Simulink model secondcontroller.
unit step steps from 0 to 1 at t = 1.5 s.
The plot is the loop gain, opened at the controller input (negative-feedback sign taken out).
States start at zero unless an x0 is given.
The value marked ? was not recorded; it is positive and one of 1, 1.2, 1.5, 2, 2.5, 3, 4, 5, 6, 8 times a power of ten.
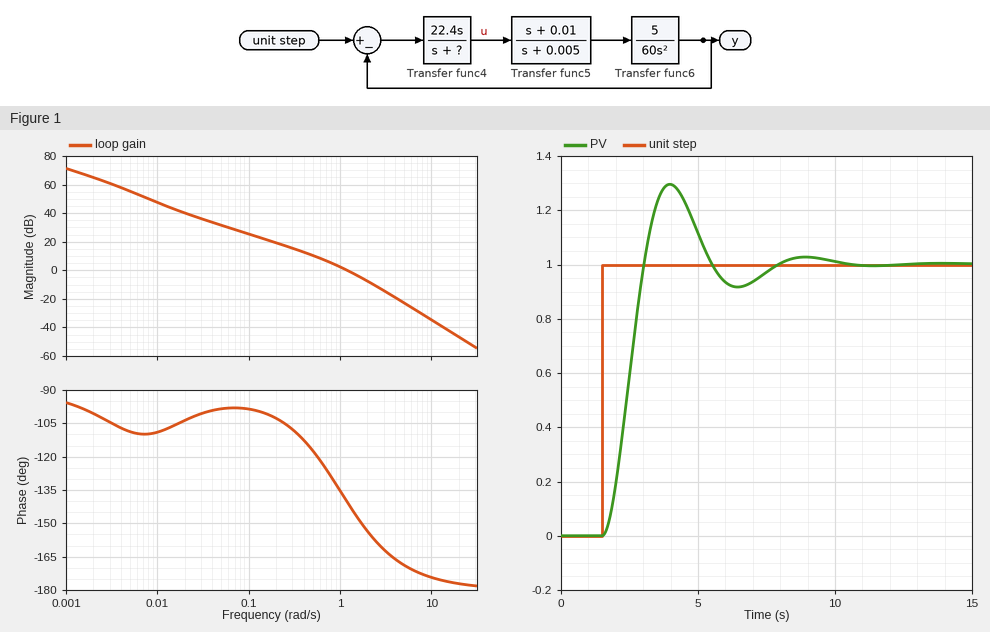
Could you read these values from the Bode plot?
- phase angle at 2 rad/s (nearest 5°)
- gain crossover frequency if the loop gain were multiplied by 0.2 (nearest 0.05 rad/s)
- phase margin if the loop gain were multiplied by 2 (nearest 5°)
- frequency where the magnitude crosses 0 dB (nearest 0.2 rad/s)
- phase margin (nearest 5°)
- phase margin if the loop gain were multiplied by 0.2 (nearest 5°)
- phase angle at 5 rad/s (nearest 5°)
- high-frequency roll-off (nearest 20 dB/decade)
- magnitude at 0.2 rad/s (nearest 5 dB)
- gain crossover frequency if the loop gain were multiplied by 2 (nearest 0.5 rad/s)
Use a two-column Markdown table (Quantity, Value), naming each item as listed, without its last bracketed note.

| Quantity | Value |
|---|---|
| phase angle at 2 rad/s | -155° |
| gain crossover frequency if the loop gain were multiplied by 0.2 | 0.35 rad/s |
| phase margin if the loop gain were multiplied by 2 | 30° |
| frequency where the magnitude crosses 0 dB | 1.2 rad/s |
| phase margin | 40° |
| phase margin if the loop gain were multiplied by 0.2 | 70° |
| phase angle at 5 rad/s | -170° |
| high-frequency roll-off | -40 dB/decade |
| magnitude at 0.2 rad/s | 20 dB |
| gain crossover frequency if the loop gain were multiplied by 2 | 2.0 rad/s |
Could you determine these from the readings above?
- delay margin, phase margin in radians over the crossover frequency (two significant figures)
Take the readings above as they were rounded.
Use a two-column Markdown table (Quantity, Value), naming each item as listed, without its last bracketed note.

| Quantity | Value |
|---|---|
| delay margin, phase margin in radians over the crossover frequency | 0.58 s |
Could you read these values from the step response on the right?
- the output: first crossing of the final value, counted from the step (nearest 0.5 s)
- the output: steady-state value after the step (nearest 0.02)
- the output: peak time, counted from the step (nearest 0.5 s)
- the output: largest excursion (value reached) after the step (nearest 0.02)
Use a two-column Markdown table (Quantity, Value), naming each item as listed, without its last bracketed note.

| Quantity | Value |
|---|---|
| the output: first crossing of the final value, counted from the step | 1.5 s |
| the output: steady-state value after the step | 1.00 |
| the output: peak time, counted from the step | 2.5 s |
| the output: largest excursion (value reached) after the step | 1.30 |
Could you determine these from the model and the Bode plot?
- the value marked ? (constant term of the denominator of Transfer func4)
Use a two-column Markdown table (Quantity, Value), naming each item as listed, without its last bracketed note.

| Quantity | Value |
|---|---|
| the value marked ? | 1 |
